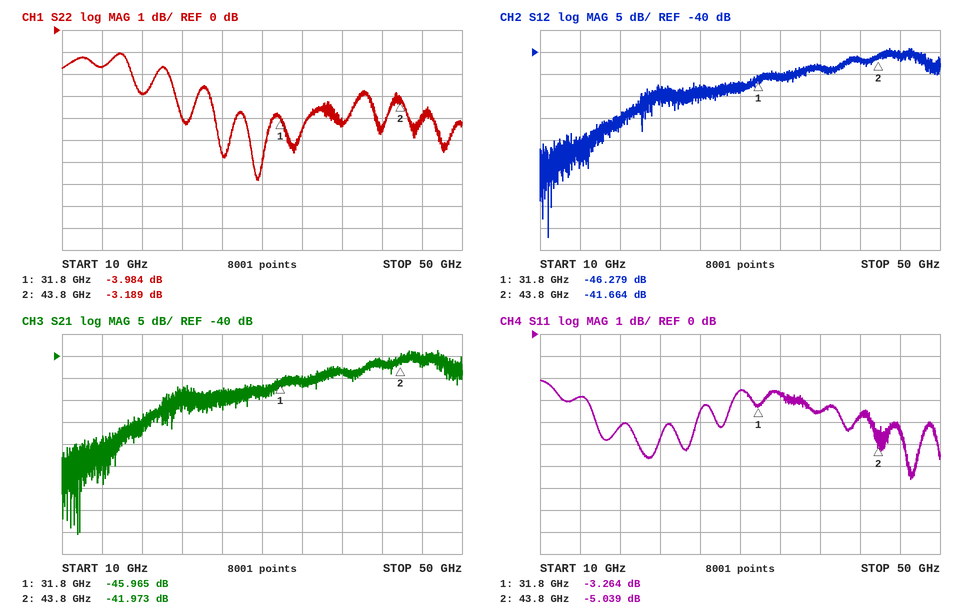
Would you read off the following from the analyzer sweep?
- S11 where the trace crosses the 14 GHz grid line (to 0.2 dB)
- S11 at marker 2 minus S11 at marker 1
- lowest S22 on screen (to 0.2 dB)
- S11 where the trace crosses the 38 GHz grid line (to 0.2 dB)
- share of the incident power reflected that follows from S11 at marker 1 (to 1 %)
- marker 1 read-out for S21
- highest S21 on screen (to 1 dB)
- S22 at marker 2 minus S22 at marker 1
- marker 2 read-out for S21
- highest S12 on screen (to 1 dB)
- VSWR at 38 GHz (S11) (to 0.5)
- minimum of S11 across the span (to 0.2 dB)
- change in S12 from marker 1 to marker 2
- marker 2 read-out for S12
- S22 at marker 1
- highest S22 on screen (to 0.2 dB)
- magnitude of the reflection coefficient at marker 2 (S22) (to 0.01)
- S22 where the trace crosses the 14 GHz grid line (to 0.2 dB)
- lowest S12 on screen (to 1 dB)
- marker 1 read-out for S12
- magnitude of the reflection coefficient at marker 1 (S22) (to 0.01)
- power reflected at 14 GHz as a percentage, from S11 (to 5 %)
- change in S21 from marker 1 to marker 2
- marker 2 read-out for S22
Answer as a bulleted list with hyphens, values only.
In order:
- -2.8 dB
- -1.775 dB
- -6.8 dB
- -3.6 dB
- 47 %
- -45.965 dB
- -39 dB
- 0.795 dB
- -41.973 dB
- -39 dB
- 5.0
- -6.6 dB
- 4.615 dB
- -41.664 dB
- -3.984 dB
- -1.0 dB
- 0.69
- -1.6 dB
- -82 dB
- -46.279 dB
- 0.63
- 50 %
- 3.992 dB
- -3.189 dB
